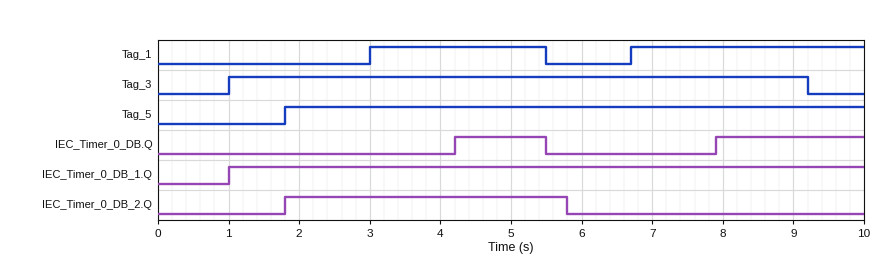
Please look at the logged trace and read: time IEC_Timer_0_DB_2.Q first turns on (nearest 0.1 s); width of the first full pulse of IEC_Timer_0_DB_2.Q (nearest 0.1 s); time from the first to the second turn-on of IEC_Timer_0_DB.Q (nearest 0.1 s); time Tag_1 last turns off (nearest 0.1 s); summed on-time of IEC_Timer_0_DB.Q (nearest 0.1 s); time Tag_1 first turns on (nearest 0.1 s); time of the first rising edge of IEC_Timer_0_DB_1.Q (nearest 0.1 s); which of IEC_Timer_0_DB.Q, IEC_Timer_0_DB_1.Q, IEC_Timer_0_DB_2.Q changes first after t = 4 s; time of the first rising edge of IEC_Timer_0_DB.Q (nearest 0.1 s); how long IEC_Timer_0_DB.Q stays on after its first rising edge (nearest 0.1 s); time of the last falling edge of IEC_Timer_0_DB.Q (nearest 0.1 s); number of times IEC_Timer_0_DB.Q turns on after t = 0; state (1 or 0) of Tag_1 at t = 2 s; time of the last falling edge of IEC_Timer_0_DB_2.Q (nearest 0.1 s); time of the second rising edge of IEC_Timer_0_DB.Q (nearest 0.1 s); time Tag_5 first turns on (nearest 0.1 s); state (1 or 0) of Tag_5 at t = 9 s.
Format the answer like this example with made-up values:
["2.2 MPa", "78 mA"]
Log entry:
["1.8 s", "4.0 s", "3.7 s", "5.5 s", "3.4 s", "3.0 s", "1.0 s", "IEC_Timer_0_DB.Q", "4.2 s", "1.3 s", "5.5 s", "2", "0", "5.8 s", "7.9 s", "1.8 s", "1"]
